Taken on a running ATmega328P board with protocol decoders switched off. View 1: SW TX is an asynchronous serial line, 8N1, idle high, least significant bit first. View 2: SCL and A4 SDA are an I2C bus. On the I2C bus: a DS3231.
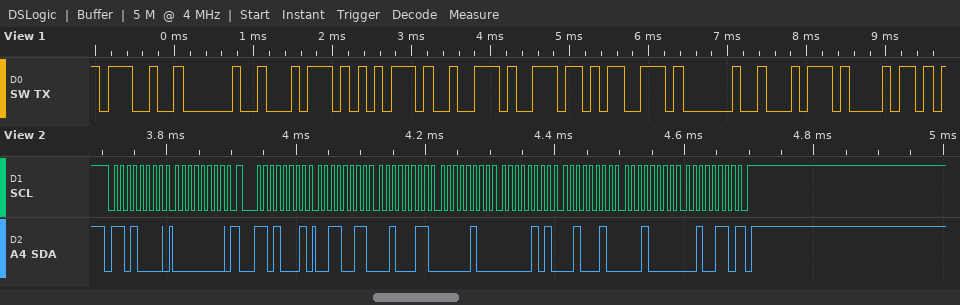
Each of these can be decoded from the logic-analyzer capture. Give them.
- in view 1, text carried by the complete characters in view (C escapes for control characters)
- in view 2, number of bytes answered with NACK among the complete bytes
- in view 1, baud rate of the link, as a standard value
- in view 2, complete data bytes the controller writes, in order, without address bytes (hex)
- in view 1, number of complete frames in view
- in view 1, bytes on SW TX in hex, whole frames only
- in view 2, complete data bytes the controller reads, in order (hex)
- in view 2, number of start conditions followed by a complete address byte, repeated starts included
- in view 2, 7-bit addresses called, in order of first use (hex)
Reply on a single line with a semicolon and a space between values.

"' turns th"; 1; 9600 baud; 00; 10; 27 20 74 75 72 6E 73 20 74 68; 33 23 04 05 22 10 26; 2; 0x68
